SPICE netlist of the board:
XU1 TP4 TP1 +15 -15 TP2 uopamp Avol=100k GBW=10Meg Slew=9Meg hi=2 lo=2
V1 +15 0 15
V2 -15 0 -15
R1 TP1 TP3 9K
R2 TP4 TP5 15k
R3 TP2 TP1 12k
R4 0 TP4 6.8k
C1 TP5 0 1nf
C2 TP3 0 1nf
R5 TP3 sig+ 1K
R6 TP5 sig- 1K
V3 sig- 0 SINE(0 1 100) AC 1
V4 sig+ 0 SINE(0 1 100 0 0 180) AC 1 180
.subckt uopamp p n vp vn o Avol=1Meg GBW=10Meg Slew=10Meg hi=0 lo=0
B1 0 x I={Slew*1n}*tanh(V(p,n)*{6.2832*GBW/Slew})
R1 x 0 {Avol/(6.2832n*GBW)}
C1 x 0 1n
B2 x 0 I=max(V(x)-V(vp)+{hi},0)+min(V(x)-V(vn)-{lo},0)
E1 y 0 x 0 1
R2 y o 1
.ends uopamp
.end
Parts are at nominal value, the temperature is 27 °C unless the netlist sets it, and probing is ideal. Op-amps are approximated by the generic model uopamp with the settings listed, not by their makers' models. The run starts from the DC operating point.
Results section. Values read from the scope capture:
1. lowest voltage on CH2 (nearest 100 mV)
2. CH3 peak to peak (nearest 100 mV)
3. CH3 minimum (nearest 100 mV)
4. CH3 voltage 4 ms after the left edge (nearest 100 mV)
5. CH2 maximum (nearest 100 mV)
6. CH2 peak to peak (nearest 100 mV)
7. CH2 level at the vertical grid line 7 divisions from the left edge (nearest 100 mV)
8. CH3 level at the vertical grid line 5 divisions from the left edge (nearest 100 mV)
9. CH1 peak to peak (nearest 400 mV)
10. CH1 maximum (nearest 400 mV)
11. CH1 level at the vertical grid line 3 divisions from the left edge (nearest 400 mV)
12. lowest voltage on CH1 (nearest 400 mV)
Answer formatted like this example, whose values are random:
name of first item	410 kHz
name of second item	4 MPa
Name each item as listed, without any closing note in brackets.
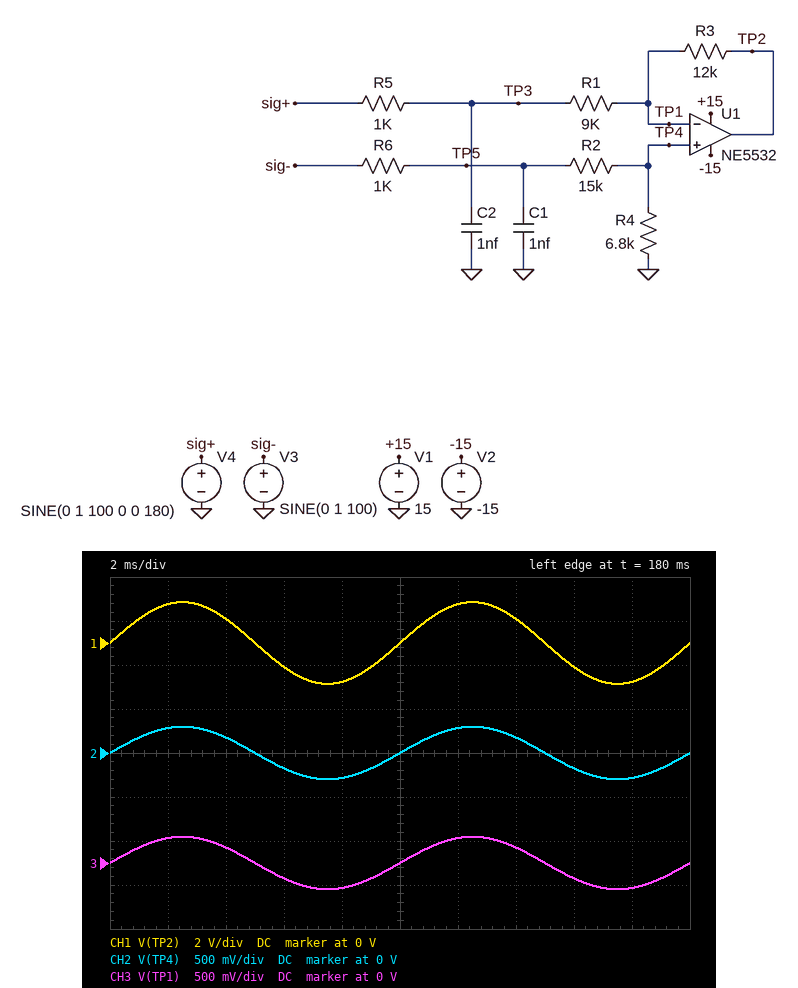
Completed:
lowest voltage on CH2	-300 mV
CH3 peak to peak	600 mV
CH3 minimum	-300 mV
CH3 voltage 4 ms after the left edge	200 mV
CH2 maximum	300 mV
CH2 peak to peak	600 mV
CH2 level at the vertical grid line 7 divisions from the left edge	200 mV
CH3 level at the vertical grid line 5 divisions from the left edge	0 V
CH1 peak to peak	3.6 V
CH1 maximum	2.0 V
CH1 level at the vertical grid line 3 divisions from the left edge	-1.2 V
lowest voltage on CH1	-2.0 V
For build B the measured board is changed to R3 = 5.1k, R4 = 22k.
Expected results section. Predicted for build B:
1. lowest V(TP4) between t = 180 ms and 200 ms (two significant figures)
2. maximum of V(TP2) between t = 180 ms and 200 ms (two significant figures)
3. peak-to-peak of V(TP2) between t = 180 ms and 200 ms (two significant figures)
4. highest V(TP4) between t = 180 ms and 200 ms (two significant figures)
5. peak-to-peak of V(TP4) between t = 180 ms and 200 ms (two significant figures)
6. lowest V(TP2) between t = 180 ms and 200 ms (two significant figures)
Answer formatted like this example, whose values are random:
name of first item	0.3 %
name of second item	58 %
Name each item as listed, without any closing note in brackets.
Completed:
lowest V(TP4) between t = 180 ms and 200 ms	-580 mV
maximum of V(TP2) between t = 180 ms and 200 ms	1.4 V
peak-to-peak of V(TP2) between t = 180 ms and 200 ms	2.8 V
highest V(TP4) between t = 180 ms and 200 ms	580 mV
peak-to-peak of V(TP4) between t = 180 ms and 200 ms	1.2 V
lowest V(TP2) between t = 180 ms and 200 ms	-1.4 V
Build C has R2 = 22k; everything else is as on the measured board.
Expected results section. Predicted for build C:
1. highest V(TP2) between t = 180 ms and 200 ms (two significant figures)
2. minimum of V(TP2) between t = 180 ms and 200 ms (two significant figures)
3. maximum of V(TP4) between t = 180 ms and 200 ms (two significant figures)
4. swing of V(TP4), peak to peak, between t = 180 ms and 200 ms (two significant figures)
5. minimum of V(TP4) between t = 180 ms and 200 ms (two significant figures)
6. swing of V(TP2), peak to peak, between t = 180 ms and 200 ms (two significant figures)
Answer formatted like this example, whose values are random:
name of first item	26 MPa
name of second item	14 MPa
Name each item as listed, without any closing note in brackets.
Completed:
highest V(TP2) between t = 180 ms and 200 ms	1.7 V
minimum of V(TP2) between t = 180 ms and 200 ms	-1.7 V
maximum of V(TP4) between t = 180 ms and 200 ms	230 mV
swing of V(TP4), peak to peak, between t = 180 ms and 200 ms	460 mV
minimum of V(TP4) between t = 180 ms and 200 ms	-230 mV
swing of V(TP2), peak to peak, between t = 180 ms and 200 ms	3.4 V
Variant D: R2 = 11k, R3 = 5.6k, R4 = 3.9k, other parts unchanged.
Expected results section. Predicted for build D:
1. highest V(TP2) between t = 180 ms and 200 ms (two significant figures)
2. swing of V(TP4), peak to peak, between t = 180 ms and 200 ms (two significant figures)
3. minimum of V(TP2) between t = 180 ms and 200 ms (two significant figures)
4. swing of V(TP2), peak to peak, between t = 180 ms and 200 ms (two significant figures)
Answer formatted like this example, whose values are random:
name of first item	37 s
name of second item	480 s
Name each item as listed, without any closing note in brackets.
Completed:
highest V(TP2) between t = 180 ms and 200 ms	940 mV
swing of V(TP4), peak to peak, between t = 180 ms and 200 ms	490 mV
minimum of V(TP2) between t = 180 ms and 200 ms	-940 mV
swing of V(TP2), peak to peak, between t = 180 ms and 200 ms	1.9 V
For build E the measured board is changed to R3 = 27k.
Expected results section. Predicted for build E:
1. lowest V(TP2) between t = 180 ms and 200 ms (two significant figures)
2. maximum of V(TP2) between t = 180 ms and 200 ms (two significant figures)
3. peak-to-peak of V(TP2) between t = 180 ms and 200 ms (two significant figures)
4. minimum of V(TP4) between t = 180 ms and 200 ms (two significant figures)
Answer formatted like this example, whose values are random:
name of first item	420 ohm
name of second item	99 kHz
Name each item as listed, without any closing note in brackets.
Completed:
lowest V(TP2) between t = 180 ms and 200 ms	-3.8 V
maximum of V(TP2) between t = 180 ms and 200 ms	3.8 V
peak-to-peak of V(TP2) between t = 180 ms and 200 ms	7.6 V
minimum of V(TP4) between t = 180 ms and 200 ms	-300 mV
